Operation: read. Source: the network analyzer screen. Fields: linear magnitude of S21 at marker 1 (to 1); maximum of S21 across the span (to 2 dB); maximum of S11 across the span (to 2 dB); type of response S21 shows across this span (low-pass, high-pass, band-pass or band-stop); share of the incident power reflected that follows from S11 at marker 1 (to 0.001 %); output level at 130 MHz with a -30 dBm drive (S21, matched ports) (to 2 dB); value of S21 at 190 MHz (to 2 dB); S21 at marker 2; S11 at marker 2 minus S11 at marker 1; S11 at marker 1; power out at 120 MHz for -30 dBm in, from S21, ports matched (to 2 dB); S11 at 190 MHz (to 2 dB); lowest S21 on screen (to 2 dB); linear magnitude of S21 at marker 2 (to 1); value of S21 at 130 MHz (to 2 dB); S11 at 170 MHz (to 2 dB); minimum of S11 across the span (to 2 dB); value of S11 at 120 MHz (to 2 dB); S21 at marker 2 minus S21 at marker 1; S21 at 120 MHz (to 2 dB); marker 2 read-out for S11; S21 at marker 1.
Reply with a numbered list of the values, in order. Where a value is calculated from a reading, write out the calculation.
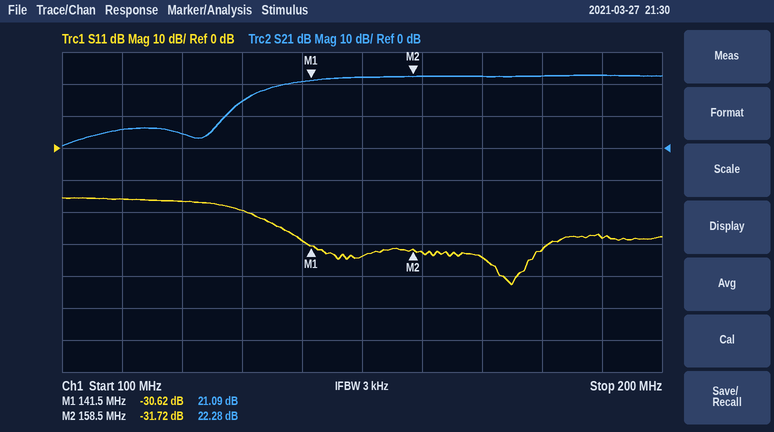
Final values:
1. 10^(21.09/20) ≈ 11
2. 22 dB
3. -16 dB
4. high-pass
5. 10^(-30.62/10) ≈ 0.087 %
6. -30 dBm + (14 dB) = -16 dBm
7. 22 dB
8. 22.28 dB
9. -31.72 − (-30.62) = -1.10 dB
10. -30.62 dB
11. -30 dBm + (4 dB) = -26 dBm
12. -28 dB
13. 0 dB
14. 10^(22.28/20) ≈ 13
15. 14 dB
16. -34 dB
17. -42 dB
18. -16 dB
19. 22.28 − (21.09) = 1.19 dB
20. 4 dB
21. -31.72 dB
22. 21.09 dB
